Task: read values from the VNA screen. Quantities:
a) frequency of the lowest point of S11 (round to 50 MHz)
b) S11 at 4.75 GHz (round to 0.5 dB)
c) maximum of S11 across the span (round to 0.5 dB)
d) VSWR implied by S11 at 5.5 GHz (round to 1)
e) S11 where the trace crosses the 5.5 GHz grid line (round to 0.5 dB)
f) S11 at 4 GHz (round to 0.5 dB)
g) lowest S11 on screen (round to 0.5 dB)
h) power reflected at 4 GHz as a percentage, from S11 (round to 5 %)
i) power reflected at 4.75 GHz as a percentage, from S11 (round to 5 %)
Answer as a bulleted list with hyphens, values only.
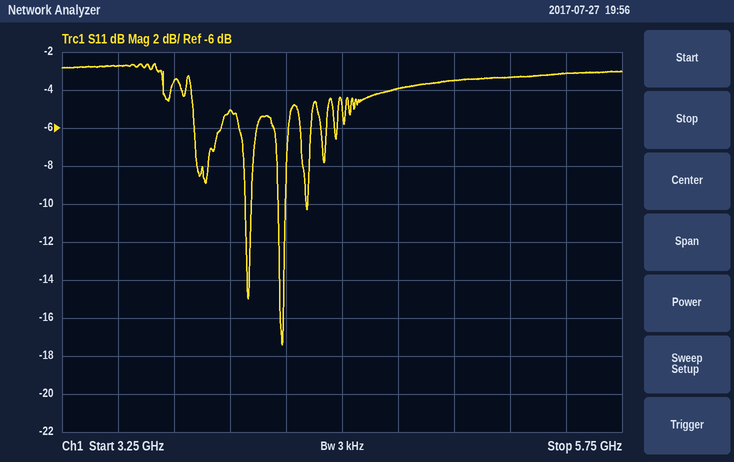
- 4.25 GHz
- -4.0 dB
- -2.5 dB
- 6
- -3.0 dB
- -5.0 dB
- -17.5 dB
- 30 %
- 40 %
